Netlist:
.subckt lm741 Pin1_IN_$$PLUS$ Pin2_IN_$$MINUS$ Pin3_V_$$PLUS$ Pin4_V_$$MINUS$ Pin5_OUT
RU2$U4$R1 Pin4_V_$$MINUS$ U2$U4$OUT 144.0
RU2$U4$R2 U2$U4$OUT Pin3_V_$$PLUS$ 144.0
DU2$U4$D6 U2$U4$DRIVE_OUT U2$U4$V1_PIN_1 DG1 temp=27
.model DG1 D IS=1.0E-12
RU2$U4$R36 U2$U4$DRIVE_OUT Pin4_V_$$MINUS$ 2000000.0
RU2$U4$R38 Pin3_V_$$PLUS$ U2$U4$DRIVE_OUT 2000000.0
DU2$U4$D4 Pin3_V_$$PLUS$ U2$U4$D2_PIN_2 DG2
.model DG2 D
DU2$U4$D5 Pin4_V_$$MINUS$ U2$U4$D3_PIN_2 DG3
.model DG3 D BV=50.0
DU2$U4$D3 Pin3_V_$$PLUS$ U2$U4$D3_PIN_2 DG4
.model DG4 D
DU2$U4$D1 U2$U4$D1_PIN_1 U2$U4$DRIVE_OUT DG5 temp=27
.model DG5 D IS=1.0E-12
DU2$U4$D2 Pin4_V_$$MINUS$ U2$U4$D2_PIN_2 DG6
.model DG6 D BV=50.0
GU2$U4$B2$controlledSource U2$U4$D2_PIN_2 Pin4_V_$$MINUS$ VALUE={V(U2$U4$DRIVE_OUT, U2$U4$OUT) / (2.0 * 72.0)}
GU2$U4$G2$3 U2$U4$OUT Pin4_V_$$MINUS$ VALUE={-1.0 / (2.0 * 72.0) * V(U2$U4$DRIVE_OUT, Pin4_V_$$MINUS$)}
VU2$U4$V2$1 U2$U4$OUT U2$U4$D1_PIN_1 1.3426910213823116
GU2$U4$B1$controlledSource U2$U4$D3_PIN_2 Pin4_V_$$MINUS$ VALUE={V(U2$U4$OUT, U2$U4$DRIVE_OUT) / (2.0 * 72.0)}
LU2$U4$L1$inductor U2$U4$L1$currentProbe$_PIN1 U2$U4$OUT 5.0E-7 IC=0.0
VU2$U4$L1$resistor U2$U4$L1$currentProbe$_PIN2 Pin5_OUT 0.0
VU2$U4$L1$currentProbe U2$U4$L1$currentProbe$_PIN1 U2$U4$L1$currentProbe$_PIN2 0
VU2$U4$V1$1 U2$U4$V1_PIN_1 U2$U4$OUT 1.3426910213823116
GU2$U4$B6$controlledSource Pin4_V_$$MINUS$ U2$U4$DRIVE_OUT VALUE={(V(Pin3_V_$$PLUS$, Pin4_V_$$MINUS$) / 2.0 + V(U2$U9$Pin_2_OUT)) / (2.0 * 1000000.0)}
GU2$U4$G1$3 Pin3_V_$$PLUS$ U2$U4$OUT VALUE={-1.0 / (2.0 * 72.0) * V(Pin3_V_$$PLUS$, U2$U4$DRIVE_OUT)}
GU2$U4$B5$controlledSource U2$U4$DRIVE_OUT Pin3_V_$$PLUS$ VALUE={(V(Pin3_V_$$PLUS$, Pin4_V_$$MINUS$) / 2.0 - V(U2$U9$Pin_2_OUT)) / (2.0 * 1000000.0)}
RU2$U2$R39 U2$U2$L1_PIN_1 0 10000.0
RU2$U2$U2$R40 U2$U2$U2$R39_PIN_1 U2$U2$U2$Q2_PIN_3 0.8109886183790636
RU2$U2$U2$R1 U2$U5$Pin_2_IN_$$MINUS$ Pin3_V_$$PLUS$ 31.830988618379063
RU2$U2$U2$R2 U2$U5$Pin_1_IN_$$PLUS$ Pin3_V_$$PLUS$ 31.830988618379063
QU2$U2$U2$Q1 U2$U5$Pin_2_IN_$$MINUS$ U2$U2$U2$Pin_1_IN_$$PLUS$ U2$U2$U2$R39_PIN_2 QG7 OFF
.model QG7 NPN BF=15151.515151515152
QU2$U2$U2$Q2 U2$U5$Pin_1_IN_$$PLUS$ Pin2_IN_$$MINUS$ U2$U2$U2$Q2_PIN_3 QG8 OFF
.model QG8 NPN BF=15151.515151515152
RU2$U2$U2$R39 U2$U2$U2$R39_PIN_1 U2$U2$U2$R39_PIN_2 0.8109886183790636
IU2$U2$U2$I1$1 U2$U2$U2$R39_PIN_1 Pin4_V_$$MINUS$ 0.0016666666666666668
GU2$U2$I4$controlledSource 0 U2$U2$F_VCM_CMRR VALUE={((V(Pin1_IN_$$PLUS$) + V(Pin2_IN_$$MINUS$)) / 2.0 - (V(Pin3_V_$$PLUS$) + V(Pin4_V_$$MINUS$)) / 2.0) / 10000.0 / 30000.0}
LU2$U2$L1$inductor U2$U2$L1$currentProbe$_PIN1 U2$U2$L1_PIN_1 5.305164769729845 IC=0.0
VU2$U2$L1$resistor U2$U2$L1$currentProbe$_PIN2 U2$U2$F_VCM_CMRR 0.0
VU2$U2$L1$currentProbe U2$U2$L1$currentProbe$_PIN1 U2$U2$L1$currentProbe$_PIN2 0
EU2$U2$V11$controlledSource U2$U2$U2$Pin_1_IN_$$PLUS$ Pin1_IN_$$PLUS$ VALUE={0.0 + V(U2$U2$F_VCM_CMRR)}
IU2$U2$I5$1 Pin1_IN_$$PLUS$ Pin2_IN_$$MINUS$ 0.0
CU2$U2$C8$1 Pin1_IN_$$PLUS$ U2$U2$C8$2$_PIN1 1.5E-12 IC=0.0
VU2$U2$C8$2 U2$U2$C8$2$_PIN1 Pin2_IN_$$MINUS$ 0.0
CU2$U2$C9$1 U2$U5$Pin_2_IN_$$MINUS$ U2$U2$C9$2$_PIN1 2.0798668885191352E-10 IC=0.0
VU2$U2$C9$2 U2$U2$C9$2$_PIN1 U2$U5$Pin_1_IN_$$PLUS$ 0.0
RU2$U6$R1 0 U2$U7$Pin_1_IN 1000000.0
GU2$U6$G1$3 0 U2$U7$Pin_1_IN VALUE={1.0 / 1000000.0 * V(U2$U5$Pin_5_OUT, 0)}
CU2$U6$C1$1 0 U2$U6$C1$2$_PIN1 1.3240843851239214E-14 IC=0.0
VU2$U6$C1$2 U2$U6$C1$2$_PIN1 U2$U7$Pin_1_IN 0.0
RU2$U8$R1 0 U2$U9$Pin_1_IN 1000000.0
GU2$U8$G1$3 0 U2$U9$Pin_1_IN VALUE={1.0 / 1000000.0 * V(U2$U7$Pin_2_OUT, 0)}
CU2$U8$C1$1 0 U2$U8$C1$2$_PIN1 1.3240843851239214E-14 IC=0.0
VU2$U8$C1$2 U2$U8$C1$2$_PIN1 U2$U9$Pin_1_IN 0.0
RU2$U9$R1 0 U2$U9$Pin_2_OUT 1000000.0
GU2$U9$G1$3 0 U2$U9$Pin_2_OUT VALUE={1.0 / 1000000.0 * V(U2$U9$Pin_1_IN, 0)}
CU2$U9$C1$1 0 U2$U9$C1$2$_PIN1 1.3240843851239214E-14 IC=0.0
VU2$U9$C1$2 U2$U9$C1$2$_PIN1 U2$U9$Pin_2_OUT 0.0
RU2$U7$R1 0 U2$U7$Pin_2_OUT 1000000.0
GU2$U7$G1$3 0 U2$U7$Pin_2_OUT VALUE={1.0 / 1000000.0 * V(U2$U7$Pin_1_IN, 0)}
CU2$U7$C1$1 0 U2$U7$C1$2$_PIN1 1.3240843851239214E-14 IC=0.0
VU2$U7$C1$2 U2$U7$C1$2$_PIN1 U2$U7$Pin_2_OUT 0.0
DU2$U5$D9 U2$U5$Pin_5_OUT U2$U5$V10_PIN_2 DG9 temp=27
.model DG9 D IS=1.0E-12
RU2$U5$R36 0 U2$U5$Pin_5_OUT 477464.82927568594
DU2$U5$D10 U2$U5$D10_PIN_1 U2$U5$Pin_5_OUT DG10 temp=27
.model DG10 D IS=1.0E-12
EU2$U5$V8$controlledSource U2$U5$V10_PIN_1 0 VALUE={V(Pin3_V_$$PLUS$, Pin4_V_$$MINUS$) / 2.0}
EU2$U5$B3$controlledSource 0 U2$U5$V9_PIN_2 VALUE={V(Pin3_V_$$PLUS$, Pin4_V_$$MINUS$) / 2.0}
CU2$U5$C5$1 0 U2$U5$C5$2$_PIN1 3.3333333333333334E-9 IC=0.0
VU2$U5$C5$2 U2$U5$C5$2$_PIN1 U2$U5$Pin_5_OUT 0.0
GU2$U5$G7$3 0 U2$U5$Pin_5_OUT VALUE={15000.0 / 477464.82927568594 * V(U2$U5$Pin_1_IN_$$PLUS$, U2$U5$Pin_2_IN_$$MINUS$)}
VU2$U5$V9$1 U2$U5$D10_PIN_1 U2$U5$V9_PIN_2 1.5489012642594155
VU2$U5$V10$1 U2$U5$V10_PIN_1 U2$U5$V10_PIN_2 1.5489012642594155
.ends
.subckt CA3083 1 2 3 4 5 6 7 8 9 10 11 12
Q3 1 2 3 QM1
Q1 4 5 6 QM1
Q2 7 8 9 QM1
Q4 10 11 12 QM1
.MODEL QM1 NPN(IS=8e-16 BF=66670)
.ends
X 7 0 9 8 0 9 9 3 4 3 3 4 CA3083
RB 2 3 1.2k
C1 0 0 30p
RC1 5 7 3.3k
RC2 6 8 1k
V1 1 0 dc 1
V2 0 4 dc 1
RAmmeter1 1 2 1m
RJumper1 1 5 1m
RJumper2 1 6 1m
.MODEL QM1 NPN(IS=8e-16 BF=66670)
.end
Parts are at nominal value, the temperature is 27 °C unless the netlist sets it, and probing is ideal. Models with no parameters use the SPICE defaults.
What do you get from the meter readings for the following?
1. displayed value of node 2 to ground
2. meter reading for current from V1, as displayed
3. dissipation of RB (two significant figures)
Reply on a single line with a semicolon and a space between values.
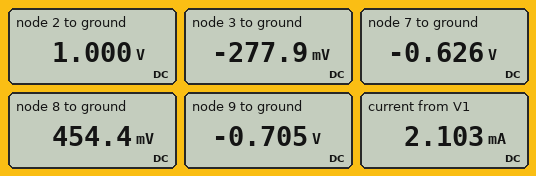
1.000 V; 2.103 mA; 1.4 mW
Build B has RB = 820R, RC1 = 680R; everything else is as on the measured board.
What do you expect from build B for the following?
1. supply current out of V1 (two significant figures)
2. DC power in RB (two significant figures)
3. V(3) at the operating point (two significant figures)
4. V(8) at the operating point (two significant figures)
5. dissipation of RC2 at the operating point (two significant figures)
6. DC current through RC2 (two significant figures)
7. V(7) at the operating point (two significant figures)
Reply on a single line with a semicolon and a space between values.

3.1 mA; 2.0 mW; -270 mV; 230 mV; 600 µW; 770 µA; 470 mV
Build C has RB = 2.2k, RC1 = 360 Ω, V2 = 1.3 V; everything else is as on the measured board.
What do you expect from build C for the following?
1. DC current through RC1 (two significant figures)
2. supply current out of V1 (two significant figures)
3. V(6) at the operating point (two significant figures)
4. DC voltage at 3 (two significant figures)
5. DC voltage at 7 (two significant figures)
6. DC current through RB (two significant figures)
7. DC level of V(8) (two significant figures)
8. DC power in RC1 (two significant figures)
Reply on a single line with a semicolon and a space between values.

360 µA; 1.4 mA; 1.0 V; -590 mV; 870 mV; 720 µA; 640 mV; 47 µW
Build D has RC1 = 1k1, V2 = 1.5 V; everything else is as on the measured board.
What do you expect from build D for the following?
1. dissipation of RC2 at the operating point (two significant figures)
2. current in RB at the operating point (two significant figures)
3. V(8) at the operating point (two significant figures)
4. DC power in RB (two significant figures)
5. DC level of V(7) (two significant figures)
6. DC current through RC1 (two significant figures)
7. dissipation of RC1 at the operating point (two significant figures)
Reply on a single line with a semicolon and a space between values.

540 µW; 1.5 mA; 260 mV; 2.6 mW; 190 mV; 740 µA; 600 µW
